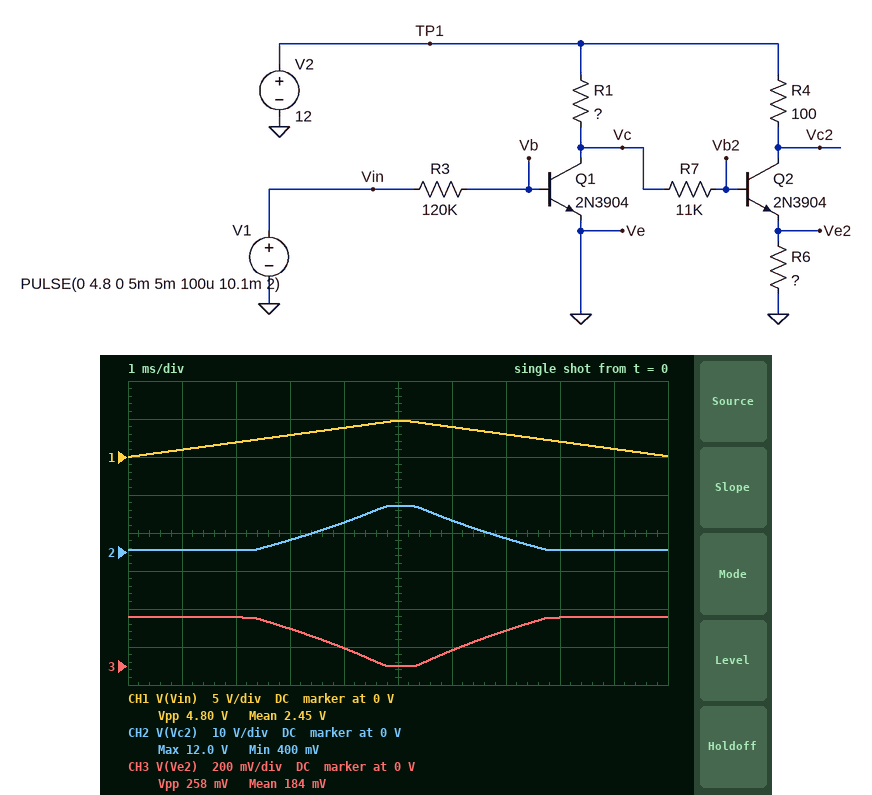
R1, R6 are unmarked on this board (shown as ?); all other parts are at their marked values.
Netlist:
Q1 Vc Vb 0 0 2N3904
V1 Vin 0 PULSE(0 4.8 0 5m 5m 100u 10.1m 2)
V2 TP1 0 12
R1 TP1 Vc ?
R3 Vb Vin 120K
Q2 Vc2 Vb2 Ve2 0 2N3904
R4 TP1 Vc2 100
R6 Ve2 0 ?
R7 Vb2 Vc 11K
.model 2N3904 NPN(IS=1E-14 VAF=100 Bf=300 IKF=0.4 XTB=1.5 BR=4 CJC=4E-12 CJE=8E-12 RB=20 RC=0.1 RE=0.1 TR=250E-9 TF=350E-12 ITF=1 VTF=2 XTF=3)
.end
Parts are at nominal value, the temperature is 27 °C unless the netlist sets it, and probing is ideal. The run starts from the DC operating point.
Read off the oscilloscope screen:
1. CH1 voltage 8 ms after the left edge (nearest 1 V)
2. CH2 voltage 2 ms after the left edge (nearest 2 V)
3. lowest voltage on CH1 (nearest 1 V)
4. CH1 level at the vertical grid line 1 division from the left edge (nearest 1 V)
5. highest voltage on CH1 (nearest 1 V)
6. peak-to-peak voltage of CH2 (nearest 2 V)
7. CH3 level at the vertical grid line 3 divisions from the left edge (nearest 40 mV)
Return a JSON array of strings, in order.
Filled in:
["2 V", "0 V", "0 V", "1 V", "5 V", "12 V", "200 mV"]
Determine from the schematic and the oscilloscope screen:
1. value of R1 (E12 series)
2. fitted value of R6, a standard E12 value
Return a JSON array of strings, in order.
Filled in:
["1.2 kΩ", "2.2 Ω"]
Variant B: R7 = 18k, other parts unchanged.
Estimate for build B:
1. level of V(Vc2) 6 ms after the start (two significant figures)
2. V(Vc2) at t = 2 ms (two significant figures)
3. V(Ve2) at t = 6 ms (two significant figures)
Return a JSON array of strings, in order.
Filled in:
["9.5 V", "2.8 V", "55 mV"]
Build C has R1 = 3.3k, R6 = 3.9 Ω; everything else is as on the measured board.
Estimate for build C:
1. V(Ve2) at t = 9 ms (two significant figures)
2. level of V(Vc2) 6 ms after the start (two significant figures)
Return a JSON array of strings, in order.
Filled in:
["440 mV", "12 V"]
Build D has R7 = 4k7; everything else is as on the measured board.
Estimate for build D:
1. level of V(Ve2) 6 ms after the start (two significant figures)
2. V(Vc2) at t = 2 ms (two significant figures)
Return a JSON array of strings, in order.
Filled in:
["150 mV", "390 mV"]
